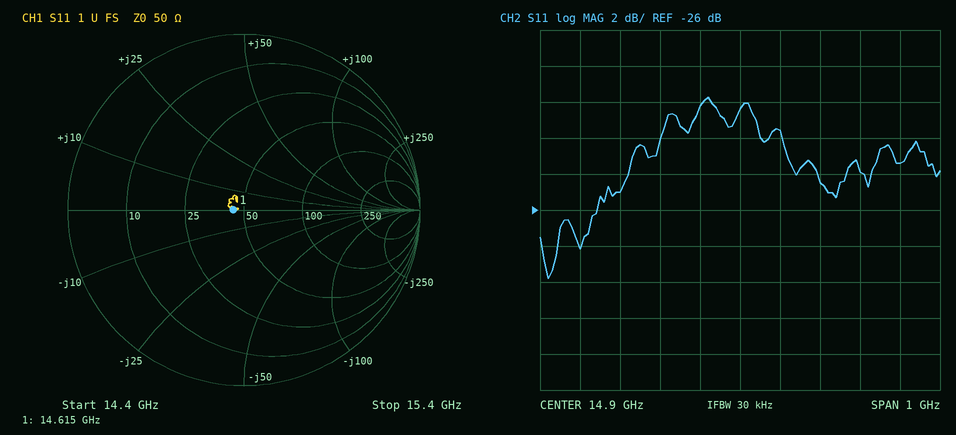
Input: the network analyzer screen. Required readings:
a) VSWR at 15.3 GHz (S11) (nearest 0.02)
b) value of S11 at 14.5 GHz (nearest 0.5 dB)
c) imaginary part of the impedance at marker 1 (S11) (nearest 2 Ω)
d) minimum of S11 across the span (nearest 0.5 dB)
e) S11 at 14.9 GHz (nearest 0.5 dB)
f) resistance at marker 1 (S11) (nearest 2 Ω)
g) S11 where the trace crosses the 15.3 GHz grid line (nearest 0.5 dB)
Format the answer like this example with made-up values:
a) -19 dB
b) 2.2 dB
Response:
a) 1.14
b) -28.0 dB
c) 0 Ω
d) -30.0 dB
e) -20.5 dB
f) 44 Ω
g) -23.5 dB
